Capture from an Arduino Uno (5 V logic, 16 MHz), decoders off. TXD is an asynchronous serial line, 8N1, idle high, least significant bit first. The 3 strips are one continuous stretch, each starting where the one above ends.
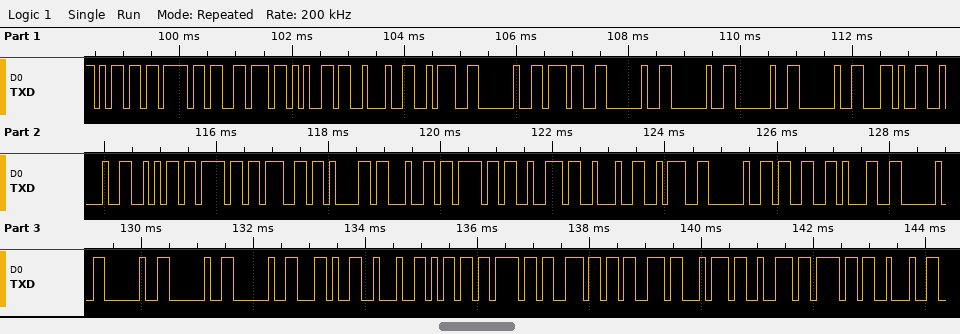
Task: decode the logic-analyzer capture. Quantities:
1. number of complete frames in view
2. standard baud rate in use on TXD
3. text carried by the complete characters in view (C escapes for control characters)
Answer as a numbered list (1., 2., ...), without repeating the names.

1. 40
2. 9600 baud
3. "move\": 7    ,\"jogador\": 31    ,\"monstro\""
